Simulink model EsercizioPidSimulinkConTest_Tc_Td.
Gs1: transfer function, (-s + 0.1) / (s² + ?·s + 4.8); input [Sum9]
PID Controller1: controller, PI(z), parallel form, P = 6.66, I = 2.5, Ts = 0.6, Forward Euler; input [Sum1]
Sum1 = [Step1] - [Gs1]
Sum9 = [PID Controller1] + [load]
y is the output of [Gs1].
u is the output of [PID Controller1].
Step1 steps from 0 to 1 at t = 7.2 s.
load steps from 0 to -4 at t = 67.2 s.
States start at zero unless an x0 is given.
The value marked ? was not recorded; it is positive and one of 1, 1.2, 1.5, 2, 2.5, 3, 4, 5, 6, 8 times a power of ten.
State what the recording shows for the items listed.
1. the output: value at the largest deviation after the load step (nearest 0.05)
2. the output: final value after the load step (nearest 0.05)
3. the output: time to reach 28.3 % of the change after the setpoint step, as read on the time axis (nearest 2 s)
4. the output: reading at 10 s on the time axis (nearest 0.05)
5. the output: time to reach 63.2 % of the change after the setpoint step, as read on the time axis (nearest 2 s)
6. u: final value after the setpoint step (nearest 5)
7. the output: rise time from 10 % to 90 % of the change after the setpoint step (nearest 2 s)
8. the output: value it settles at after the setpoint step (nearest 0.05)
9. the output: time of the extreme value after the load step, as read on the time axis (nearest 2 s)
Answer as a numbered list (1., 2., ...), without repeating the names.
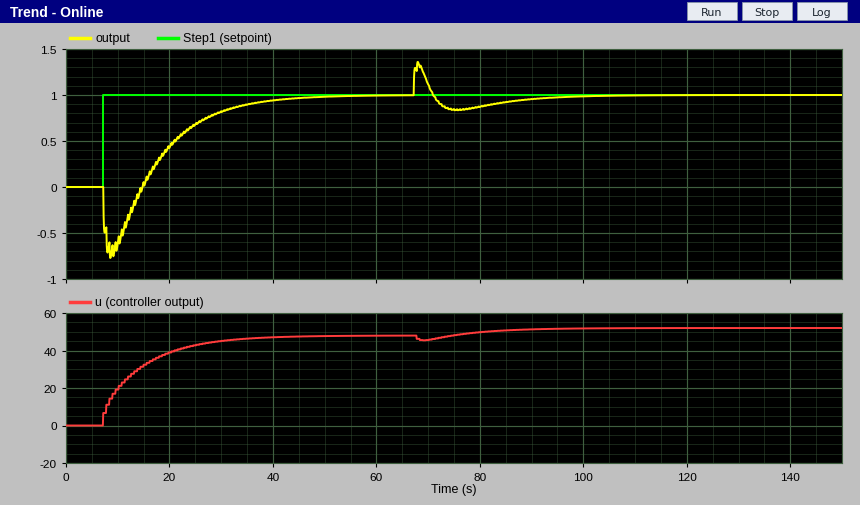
1. 1.35
2. 1.00
3. 18 s
4. -0.60
5. 24 s
6. 50
7. 20 s
8. 1.00
9. 68 s
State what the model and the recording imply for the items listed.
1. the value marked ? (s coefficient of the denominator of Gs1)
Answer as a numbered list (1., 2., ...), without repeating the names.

1. 12
